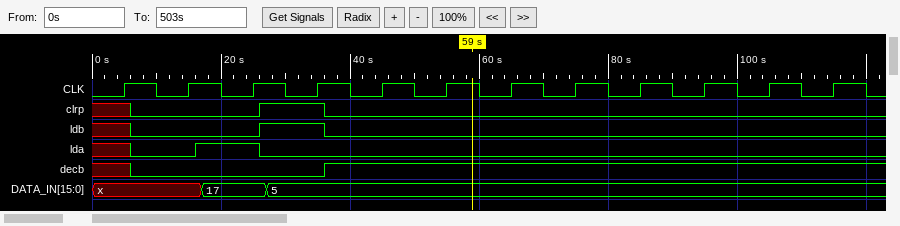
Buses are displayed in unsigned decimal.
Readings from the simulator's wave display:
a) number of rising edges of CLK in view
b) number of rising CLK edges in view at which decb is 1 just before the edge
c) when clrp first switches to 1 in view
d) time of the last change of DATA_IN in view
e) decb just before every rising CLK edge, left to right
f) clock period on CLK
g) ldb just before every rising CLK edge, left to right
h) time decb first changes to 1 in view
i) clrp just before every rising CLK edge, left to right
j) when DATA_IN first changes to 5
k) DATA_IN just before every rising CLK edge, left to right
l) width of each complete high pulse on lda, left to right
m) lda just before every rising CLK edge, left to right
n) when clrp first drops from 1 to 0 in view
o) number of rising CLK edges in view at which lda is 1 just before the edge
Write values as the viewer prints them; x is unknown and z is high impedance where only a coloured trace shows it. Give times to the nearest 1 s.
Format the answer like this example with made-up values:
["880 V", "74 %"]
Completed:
["12", "8", "26 s", "27 s", "x 0 0 0 1 1 1 1 1 1 1 1", "10 s", "x 0 0 1 0 0 0 0 0 0 0 0", "36 s", "x 0 0 1 0 0 0 0 0 0 0 0", "27 s", "x, x, 17, 5, 5, 5, 5, 5, 5, 5, 5, 5", "10 s", "x 0 1 0 0 0 0 0 0 0 0 0", "36 s", "1"]
